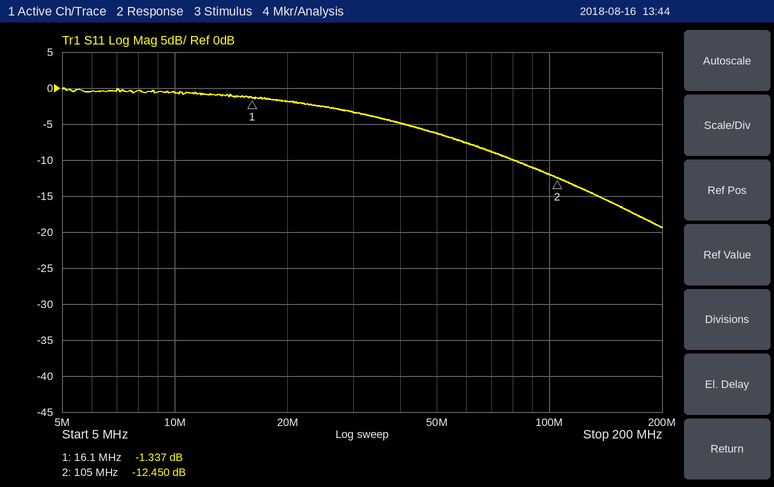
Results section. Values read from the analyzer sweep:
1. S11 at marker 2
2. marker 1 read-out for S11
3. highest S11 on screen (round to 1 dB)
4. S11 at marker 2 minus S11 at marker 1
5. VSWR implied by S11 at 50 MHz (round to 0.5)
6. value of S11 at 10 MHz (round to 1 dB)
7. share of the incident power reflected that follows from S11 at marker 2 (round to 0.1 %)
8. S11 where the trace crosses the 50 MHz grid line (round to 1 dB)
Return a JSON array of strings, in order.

["-12.450 dB", "-1.337 dB", "0 dB", "-11.113 dB", "3.0", "-1 dB", "5.7 %", "-6 dB"]
